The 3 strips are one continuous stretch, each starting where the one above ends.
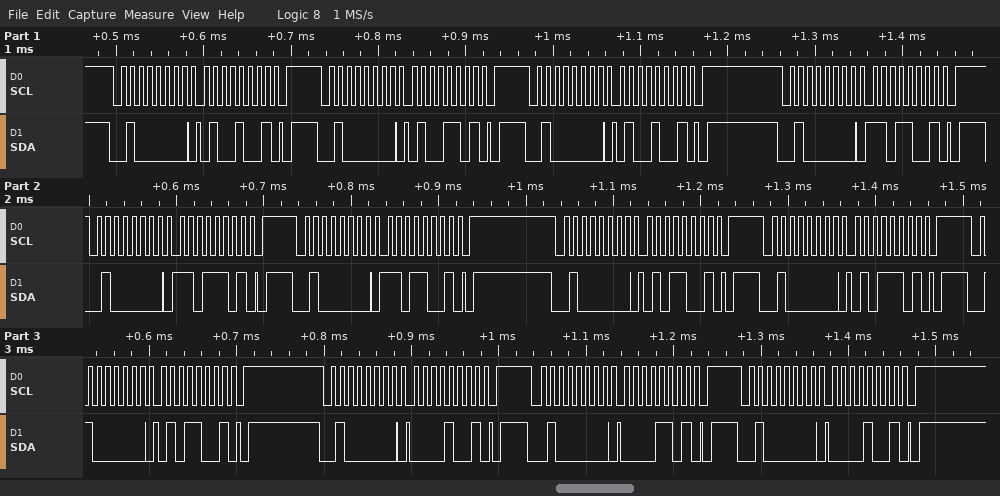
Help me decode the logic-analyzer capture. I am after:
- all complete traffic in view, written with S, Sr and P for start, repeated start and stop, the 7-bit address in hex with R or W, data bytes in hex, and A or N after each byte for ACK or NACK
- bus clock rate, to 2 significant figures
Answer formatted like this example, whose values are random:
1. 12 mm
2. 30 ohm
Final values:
1. S 20W A 49 A P S 20W A 4D A P S 20W A 49 A P S 20W A D9 A P S 20W A DD A P S 20W A D9 A P S 20W A 59 A P S 20W A 5D A P S 20W A 59 A P S 20W A 09 A P S 20W A 0D A P S 20W A 09 A P
2. 100 kHz
